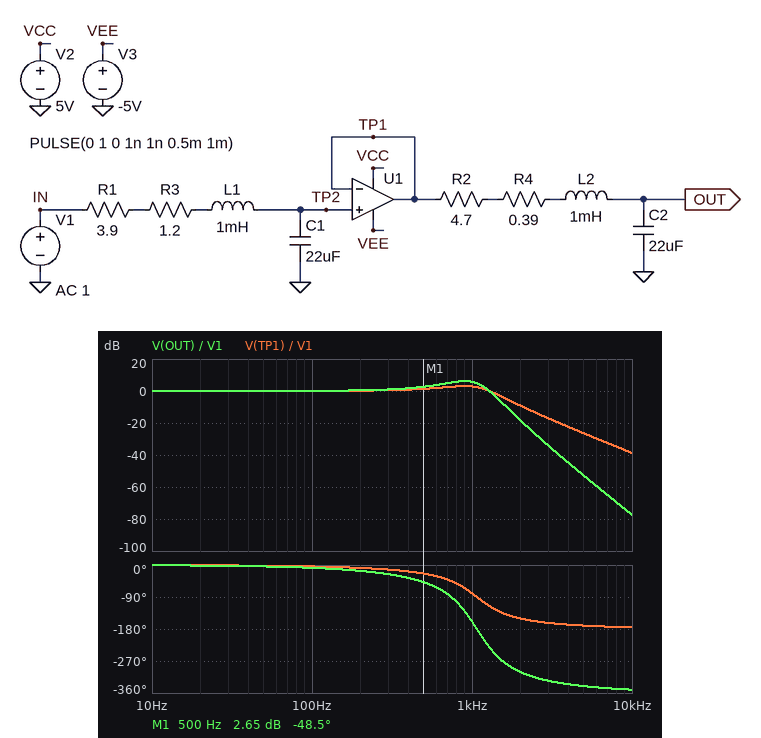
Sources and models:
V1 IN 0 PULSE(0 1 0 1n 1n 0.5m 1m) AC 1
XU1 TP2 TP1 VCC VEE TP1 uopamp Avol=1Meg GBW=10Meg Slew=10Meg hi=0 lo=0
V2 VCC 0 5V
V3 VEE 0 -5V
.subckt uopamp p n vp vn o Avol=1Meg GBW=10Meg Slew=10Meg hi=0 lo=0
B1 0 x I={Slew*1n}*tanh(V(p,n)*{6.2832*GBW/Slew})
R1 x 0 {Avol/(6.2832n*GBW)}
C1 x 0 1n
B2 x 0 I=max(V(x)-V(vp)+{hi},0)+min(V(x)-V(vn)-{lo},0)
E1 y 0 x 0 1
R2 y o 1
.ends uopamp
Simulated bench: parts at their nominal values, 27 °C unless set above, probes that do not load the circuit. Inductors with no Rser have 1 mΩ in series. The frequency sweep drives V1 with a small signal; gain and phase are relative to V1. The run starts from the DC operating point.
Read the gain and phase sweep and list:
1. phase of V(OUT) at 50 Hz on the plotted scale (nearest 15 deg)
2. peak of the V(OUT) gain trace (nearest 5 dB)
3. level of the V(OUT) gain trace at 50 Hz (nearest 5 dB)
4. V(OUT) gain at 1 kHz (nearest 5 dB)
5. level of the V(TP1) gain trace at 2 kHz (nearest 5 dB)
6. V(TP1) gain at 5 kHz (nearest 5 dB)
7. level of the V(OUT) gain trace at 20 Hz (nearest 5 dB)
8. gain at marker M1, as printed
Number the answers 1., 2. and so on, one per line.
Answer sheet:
1. 0 deg
2. 5 dB
3. 0 dB
4. 5 dB
5. -10 dB
6. -25 dB
7. 0 dB
8. 2.65 dB
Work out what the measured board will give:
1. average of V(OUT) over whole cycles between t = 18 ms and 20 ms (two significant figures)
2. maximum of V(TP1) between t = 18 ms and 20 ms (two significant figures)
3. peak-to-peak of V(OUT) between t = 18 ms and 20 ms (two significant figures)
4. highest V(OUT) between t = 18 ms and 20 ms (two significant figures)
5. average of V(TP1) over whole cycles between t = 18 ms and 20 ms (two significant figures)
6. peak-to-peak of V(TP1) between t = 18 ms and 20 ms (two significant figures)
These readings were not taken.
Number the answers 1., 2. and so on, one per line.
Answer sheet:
1. 500 mV
2. 1.4 V
3. 2.5 V
4. 1.7 V
5. 500 mV
6. 1.8 V
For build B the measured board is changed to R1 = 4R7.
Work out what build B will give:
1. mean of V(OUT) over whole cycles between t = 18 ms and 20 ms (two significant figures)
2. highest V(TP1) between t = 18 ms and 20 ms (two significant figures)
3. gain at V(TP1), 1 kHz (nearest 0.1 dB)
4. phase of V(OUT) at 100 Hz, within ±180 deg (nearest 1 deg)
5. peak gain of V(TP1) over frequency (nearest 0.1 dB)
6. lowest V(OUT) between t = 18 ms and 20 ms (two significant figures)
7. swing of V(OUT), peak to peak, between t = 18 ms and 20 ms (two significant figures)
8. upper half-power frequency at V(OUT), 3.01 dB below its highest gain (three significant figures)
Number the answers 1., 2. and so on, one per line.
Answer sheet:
1. 500 mV
2. 1.3 V
3. 1.7 dB
4. -9 deg
5. 2.1 dB
6. -580 mV
7. 2.2 V
8. 1.15 kHz
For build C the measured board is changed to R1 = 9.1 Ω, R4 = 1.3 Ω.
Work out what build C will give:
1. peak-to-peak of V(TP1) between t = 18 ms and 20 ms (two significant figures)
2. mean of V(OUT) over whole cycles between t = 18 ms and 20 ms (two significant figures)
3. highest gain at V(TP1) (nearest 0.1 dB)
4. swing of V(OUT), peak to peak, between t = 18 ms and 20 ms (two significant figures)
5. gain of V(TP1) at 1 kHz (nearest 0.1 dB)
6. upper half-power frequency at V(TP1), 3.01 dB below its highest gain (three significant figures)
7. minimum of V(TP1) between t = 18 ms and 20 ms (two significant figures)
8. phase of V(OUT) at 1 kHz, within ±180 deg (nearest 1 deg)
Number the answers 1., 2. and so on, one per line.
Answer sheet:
1. 930 mV
2. 500 mV
3. 0 dB
4. 1.1 V
5. -3.1 dB
6. 987 Hz
7. 35 mV
8. -166 deg
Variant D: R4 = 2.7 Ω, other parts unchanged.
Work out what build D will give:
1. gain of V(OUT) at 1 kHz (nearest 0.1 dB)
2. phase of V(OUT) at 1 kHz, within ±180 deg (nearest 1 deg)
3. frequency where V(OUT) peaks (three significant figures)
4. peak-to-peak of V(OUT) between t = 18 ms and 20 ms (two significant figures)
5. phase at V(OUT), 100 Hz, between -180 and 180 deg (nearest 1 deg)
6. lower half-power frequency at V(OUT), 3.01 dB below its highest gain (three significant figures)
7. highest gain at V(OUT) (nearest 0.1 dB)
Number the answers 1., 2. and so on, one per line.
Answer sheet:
1. 2.6 dB
2. -162 deg
3. 830 Hz
4. 1.7 V
5. -10 deg
6. 249 Hz
7. 3.5 dB
